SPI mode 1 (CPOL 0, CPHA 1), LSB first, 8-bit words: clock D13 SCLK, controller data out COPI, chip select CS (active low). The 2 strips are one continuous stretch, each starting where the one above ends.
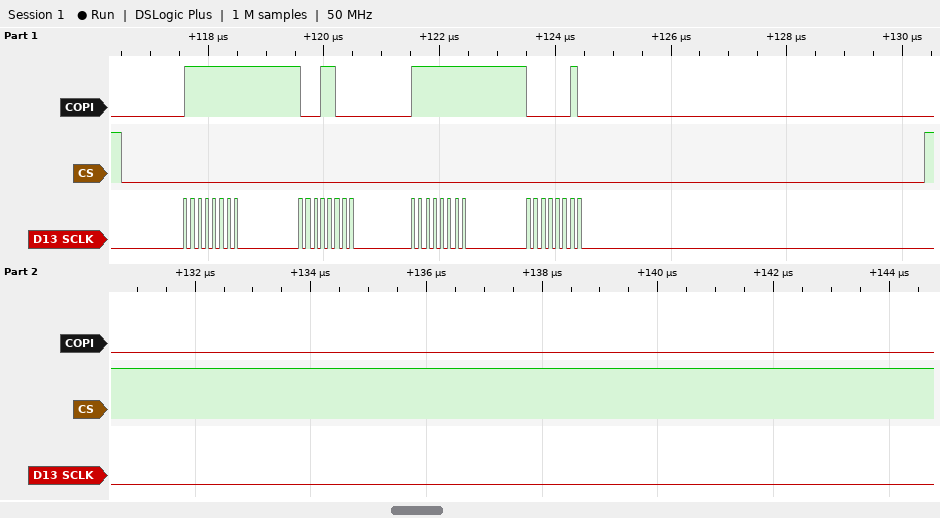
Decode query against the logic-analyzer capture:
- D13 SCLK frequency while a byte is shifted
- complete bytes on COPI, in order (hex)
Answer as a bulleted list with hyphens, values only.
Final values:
- 8 MHz
- FF 18 FF 40
